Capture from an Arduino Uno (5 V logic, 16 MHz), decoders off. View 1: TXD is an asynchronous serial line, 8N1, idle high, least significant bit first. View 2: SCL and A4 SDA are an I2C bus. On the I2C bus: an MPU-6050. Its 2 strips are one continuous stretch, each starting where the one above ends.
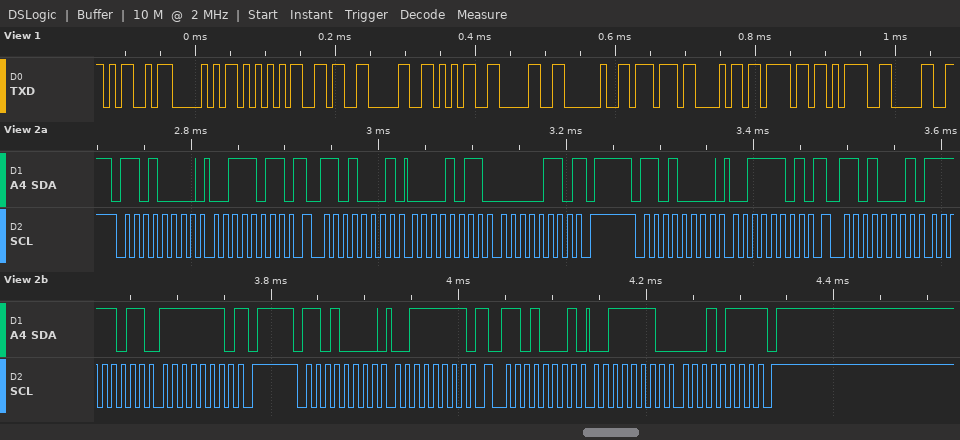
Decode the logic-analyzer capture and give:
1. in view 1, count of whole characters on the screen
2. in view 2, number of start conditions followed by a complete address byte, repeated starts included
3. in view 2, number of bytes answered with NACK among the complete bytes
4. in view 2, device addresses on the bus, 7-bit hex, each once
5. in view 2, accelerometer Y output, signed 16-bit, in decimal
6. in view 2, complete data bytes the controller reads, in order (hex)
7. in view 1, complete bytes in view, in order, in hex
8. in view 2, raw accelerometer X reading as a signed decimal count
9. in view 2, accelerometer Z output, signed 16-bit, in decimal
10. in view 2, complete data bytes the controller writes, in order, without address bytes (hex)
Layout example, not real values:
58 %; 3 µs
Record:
13; 6; 3; 0x68; -1026; 0B 06 FB FE 3E 17; 0x4D 0x50 0x55 0x36 0x30 0x35 0x30 0x20 0x77 0x68 0x6F 0x3D 0x30; 2822; 15895; 3B 3D 3F
